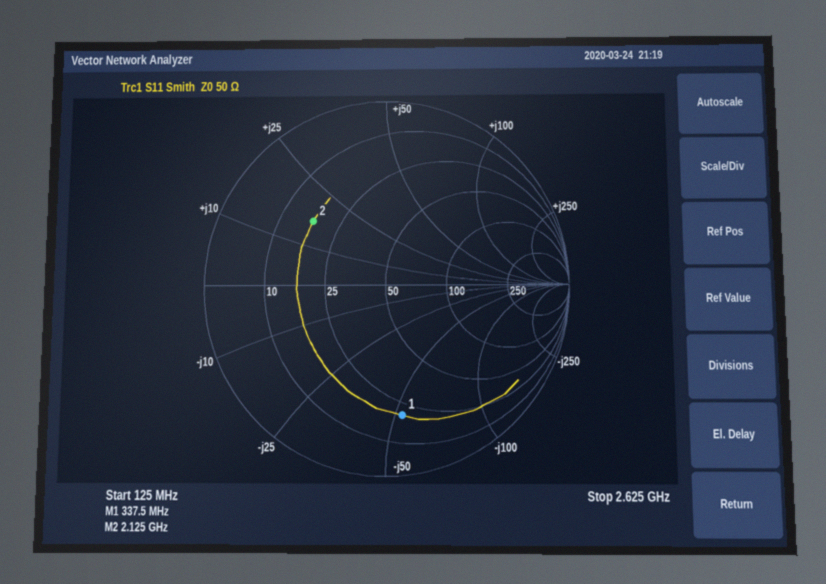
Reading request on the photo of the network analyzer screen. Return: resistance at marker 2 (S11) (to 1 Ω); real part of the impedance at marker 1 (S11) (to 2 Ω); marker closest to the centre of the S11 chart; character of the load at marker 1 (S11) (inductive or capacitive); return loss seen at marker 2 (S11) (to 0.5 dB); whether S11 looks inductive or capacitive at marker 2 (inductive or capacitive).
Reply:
17 Ω
20 Ω
marker 2
capacitive
5.5 dB
inductive
